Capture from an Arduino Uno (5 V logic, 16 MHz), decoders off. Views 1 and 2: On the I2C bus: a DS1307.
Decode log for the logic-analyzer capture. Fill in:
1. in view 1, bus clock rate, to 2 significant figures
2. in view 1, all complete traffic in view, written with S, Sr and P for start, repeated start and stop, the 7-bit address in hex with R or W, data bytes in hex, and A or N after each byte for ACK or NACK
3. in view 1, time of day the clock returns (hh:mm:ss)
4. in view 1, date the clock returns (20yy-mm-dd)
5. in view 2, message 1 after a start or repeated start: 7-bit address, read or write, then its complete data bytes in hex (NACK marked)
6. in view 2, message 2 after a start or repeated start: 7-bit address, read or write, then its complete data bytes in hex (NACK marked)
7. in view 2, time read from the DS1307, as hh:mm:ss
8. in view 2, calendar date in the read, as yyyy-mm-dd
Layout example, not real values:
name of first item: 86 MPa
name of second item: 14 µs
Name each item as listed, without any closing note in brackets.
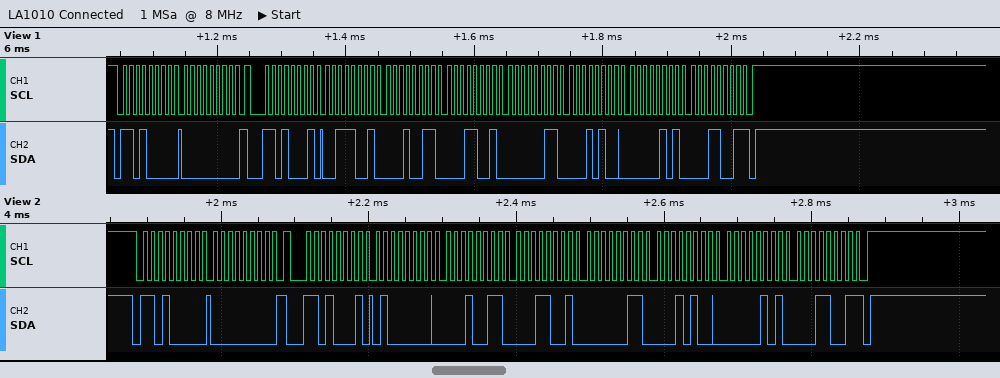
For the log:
in view 1, bus clock rate, to 2 significant figures: 100 kHz
in view 1, all complete traffic in view, written with S, Sr and P for start, repeated start and stop, the 7-bit address in hex with R or W, data bytes in hex, and A or N after each byte for ACK or NACK: S 68W A 00 A Sr 68R A 39 A 13 A 19 A 03 A 14 A 05 A 19 N P
in view 1, time of day the clock returns: 19:13:39
in view 1, date the clock returns: 2019-05-14
in view 2, message 1 after a start or repeated start: 7-bit address, read or write, then its complete data bytes in hex: 0x68 write: 00
in view 2, message 2 after a start or repeated start: 7-bit address, read or write, then its complete data bytes in hex: 0x68 read: 40 13 19 03 14 05 19 NACK
in view 2, time read from the DS1307, as hh:mm:ss: 19:13:40
in view 2, calendar date in the read, as yyyy-mm-dd: 2019-05-14
